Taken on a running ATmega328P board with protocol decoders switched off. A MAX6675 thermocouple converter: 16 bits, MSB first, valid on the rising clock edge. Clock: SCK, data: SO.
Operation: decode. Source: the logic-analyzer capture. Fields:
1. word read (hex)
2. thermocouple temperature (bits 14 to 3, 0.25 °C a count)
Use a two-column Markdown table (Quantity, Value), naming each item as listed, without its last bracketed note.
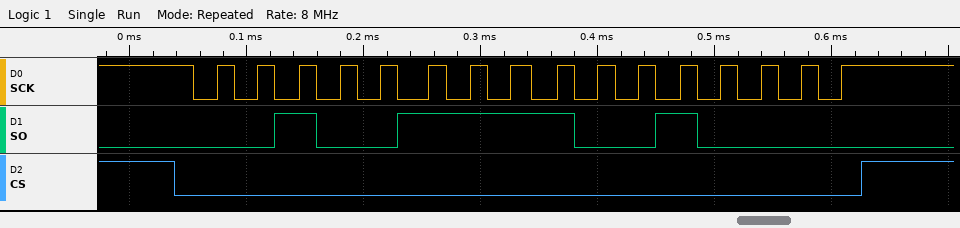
| Quantity | Value |
|---|---|
| word read | 0x2790 |
| thermocouple temperature | 316.50 °C |
